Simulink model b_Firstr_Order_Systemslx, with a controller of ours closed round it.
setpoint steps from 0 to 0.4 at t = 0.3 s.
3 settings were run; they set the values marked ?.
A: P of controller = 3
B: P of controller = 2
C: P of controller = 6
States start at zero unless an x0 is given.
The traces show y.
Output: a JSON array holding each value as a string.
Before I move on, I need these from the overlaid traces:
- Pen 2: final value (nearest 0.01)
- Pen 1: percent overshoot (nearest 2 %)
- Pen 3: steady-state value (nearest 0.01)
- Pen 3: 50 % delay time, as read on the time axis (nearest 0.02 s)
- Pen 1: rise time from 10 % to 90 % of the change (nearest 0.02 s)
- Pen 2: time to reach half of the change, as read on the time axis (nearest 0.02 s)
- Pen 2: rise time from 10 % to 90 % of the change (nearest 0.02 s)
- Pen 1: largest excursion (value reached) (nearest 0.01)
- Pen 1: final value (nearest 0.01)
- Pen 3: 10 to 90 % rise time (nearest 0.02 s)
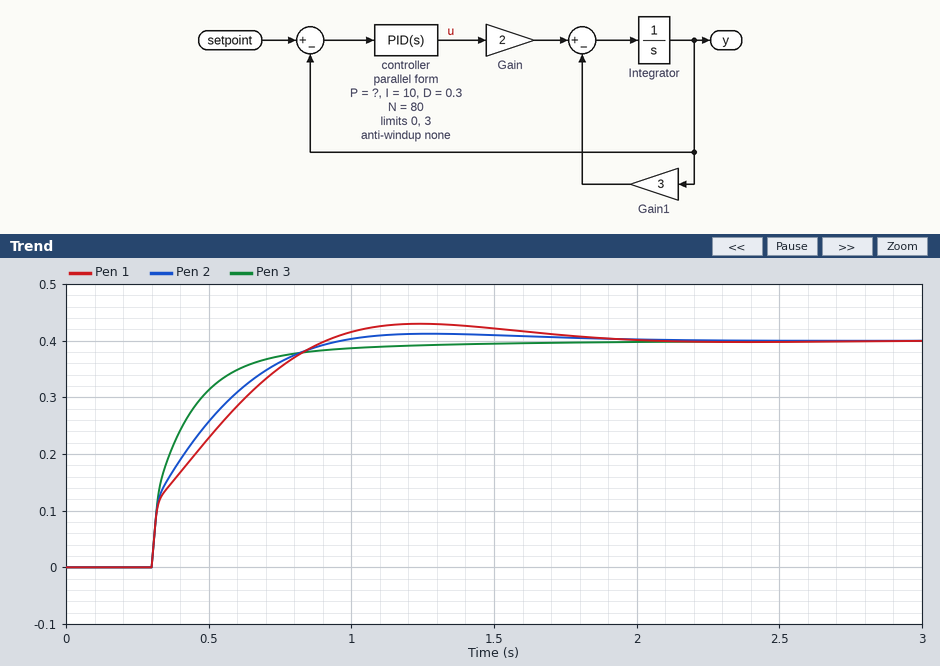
["0.40", "8 %", "0.40", "0.36 s", "0.46 s", "0.42 s", "0.44 s", "0.43", "0.40", "0.34 s"]
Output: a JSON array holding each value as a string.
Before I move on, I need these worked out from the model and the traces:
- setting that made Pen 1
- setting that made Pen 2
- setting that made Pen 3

["B", "A", "C"]
